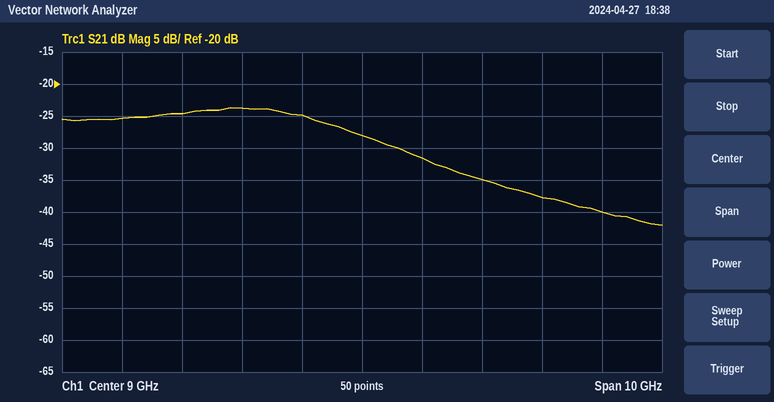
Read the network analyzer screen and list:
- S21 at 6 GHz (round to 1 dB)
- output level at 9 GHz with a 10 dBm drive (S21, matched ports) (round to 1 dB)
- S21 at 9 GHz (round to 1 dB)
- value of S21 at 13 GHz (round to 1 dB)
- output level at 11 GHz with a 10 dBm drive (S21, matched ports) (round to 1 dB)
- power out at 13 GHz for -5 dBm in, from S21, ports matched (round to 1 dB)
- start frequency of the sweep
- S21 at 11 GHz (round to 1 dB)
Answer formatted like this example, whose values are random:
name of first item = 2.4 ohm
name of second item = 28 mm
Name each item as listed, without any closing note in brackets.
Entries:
S21 at 6 GHz = -25 dB
output level at 9 GHz with a 10 dBm drive (S21, matched ports) = -18 dBm
S21 at 9 GHz = -28 dB
value of S21 at 13 GHz = -40 dB
output level at 11 GHz with a 10 dBm drive (S21, matched ports) = -25 dBm
power out at 13 GHz for -5 dBm in, from S21, ports matched = -45 dBm
start frequency of the sweep = 4 GHz
S21 at 11 GHz = -35 dB
